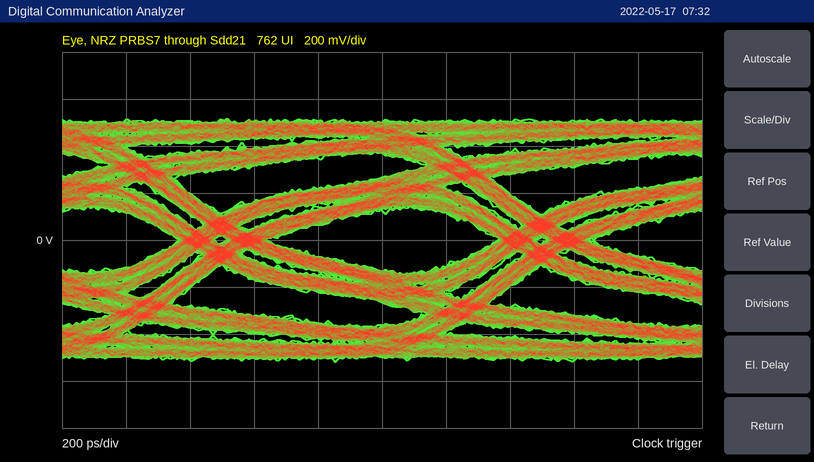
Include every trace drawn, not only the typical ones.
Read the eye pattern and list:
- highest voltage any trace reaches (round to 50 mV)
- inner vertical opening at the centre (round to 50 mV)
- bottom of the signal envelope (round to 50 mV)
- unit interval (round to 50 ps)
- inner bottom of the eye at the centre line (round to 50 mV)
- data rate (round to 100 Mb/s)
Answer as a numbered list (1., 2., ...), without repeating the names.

1. 500 mV
2. 250 mV
3. -500 mV
4. 1.00 ns
5. -150 mV
6. 1.0 Gb/s
